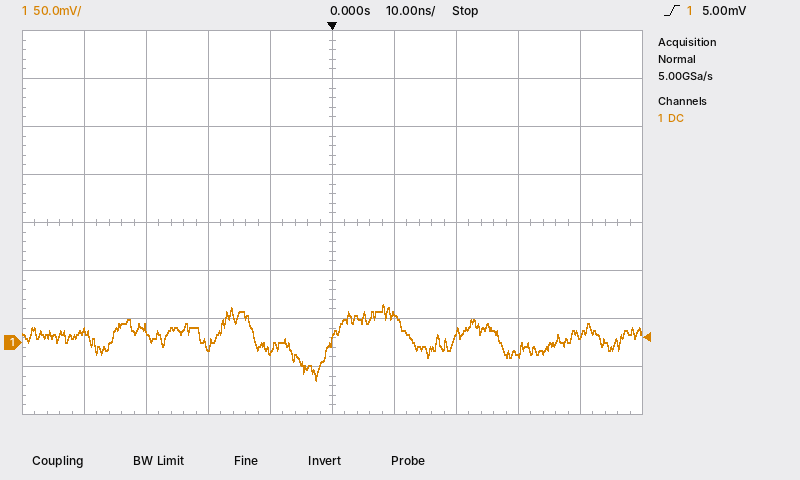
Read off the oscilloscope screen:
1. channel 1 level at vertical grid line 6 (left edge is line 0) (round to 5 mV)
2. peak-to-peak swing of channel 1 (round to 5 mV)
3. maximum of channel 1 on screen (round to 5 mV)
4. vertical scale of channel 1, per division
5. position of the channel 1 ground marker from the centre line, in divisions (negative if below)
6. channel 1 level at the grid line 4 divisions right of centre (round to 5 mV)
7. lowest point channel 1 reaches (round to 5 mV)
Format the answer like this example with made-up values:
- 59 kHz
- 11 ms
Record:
- 30 mV
- 80 mV
- 40 mV
- 50 mV
- -2.5 div
- 10 mV
- -40 mV
